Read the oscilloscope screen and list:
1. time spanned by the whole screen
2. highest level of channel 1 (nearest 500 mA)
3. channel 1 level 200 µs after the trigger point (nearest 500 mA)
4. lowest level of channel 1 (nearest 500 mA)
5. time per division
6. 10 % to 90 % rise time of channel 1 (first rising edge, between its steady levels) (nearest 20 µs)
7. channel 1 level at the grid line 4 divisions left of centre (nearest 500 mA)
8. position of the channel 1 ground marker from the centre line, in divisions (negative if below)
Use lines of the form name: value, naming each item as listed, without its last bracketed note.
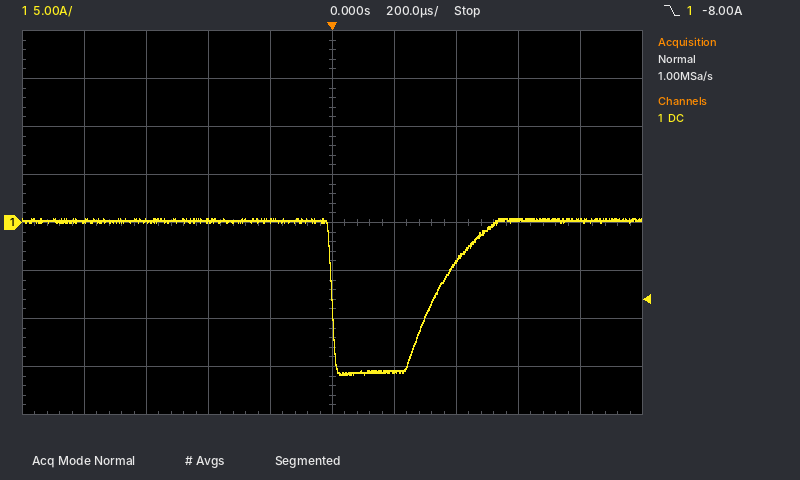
time spanned by the whole screen: 2 ms
highest level of channel 1: 500 mA
channel 1 level 200 µs after the trigger point: -15.5 A
lowest level of channel 1: -16.0 A
time per division: 200 µs
10 % to 90 % rise time of channel 1 (first rising edge, between its steady levels): 220 µs
channel 1 level at the grid line 4 divisions left of centre: 0.0 A
position of the channel 1 ground marker from the centre line, in divisions: 0.0 div
